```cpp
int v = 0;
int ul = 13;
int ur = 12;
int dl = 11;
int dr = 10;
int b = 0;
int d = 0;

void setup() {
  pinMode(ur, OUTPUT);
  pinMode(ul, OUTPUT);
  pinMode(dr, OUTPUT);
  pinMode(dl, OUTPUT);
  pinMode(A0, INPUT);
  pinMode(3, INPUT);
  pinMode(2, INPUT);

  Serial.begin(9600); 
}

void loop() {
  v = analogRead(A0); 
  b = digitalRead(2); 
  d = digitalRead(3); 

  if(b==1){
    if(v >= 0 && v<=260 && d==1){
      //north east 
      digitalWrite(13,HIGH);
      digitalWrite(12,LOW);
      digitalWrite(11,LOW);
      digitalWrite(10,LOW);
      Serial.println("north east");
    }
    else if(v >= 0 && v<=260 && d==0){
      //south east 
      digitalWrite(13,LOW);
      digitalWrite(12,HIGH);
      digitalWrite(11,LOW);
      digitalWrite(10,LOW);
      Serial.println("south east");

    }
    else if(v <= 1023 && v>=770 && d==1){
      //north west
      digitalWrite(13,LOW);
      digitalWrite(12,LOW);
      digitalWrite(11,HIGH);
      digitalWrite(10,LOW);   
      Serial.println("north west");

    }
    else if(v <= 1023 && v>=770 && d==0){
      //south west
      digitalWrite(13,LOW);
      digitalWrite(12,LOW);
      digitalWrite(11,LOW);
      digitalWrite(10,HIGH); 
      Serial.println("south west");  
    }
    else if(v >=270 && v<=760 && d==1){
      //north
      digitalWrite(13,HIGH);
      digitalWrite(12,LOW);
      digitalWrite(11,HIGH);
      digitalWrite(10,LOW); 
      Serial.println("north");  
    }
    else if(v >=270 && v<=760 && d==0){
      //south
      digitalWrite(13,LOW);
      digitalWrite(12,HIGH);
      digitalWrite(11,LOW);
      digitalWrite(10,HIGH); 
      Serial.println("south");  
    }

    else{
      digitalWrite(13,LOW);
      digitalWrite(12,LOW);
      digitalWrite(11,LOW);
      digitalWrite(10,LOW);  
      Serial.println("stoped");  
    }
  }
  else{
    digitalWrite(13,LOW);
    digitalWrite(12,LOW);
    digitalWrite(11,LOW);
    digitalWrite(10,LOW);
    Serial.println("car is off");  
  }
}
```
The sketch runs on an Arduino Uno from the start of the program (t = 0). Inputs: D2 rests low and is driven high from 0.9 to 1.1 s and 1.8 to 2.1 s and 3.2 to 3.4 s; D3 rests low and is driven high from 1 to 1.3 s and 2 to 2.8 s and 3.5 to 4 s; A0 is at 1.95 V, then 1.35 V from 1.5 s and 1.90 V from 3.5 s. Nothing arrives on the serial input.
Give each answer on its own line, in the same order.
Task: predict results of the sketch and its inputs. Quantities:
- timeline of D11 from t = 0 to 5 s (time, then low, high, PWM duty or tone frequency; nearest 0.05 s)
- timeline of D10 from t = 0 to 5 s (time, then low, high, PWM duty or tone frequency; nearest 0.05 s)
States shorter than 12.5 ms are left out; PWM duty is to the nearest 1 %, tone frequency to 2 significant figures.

0 s low; 1 s high; 1.1 s low; 2 s high; 2.1 s low
0 s low; 0.9 s high; 1 s low; 1.8 s high; 2 s low; 3.2 s high; 3.4 s low
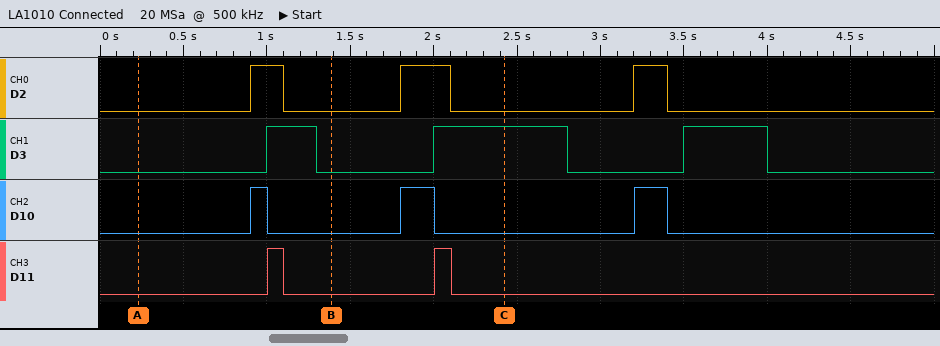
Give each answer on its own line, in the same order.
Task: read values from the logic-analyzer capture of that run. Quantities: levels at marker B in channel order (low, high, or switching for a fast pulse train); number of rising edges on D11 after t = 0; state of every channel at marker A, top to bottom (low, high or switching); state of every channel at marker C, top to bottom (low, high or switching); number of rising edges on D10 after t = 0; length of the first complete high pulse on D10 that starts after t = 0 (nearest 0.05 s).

D2 low, D3 low, D10 low, D11 low
2
D2 low, D3 low, D10 low, D11 low
D2 low, D3 high, D10 low, D11 low
3
0.10 s
